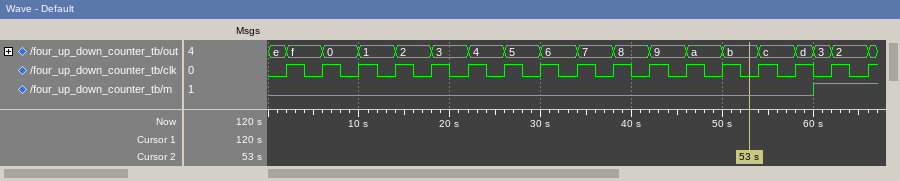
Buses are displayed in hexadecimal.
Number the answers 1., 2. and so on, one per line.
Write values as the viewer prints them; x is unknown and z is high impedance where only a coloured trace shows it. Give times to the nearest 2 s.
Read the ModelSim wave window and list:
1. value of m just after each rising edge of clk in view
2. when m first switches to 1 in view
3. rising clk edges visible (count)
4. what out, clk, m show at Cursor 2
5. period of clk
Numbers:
1. 0 0 0 0 0 0 0 0 0 0 0 0 0 0 0 1 1
2. 60 s
3. 17
4. out=b, clk=0, m=0
5. 4 s
